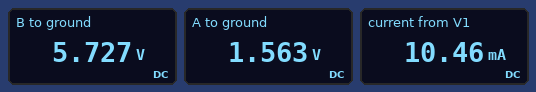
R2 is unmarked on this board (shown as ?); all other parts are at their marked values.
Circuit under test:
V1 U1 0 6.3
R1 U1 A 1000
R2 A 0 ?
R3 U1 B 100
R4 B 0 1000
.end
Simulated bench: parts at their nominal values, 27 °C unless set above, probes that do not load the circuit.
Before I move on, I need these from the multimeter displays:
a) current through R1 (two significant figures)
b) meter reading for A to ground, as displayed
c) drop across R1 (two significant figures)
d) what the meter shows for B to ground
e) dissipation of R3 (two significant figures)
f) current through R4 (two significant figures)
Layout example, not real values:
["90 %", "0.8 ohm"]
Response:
["4.7 mA", "1.563 V", "4.7 V", "5.727 V", "3.3 mW", "5.7 mA"]
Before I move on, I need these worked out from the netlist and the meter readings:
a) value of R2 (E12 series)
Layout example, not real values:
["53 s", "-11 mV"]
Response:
["330 Ω"]
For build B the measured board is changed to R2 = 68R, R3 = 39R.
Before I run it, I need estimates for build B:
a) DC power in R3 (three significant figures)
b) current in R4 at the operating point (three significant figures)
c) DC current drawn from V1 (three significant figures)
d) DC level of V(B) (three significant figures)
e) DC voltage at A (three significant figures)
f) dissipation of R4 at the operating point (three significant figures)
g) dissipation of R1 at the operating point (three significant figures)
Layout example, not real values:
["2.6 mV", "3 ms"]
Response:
["1.43 mW", "6.06 mA", "12.0 mA", "6.06 V", "401 mV", "36.8 mW", "34.8 mW"]
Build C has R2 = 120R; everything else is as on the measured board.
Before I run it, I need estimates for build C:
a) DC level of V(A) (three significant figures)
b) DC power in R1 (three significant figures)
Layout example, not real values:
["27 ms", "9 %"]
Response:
["675 mV", "31.6 mW"]
